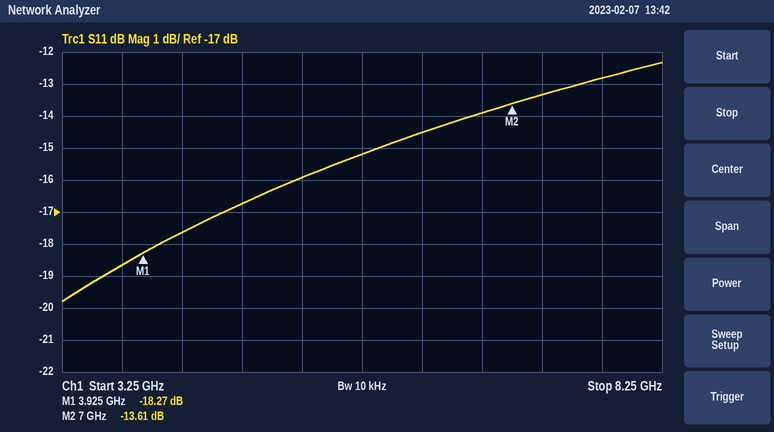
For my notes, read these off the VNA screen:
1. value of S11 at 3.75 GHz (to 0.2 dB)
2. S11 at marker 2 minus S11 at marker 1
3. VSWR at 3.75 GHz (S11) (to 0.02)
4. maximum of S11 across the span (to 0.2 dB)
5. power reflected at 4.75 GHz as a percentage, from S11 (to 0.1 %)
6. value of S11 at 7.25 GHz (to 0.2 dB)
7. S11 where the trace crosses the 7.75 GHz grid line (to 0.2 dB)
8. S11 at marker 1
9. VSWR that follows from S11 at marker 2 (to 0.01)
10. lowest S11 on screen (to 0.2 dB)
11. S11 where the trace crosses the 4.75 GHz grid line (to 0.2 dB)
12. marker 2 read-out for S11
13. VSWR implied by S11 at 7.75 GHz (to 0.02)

-18.6 dB
4.66 dB
1.26
-12.4 dB
2.1 %
-13.4 dB
-12.8 dB
-18.27 dB
1.53
-19.8 dB
-16.8 dB
-13.61 dB
1.60
